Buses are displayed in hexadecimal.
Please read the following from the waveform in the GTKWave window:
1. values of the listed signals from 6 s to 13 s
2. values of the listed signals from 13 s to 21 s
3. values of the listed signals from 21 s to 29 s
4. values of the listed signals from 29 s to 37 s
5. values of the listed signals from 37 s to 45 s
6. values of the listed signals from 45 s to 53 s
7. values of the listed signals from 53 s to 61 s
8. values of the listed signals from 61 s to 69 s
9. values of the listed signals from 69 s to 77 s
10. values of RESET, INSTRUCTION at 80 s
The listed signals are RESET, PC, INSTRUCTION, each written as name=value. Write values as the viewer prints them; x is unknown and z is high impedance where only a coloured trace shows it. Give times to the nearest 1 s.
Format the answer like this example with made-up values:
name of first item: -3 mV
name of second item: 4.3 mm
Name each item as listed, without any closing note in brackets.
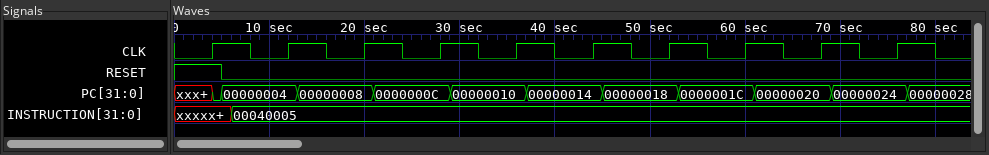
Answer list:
values of the listed signals from 6 s to 13 s: RESET=0, PC=00000004, INSTRUCTION=00040005
values of the listed signals from 13 s to 21 s: RESET=0, PC=00000008, INSTRUCTION=00040005
values of the listed signals from 21 s to 29 s: RESET=0, PC=0000000C, INSTRUCTION=00040005
values of the listed signals from 29 s to 37 s: RESET=0, PC=00000010, INSTRUCTION=00040005
values of the listed signals from 37 s to 45 s: RESET=0, PC=00000014, INSTRUCTION=00040005
values of the listed signals from 45 s to 53 s: RESET=0, PC=00000018, INSTRUCTION=00040005
values of the listed signals from 53 s to 61 s: RESET=0, PC=0000001C, INSTRUCTION=00040005
values of the listed signals from 61 s to 69 s: RESET=0, PC=00000020, INSTRUCTION=00040005
values of the listed signals from 69 s to 77 s: RESET=0, PC=00000024, INSTRUCTION=00040005
values of RESET, INSTRUCTION at 80 s: RESET=0, INSTRUCTION=00040005
